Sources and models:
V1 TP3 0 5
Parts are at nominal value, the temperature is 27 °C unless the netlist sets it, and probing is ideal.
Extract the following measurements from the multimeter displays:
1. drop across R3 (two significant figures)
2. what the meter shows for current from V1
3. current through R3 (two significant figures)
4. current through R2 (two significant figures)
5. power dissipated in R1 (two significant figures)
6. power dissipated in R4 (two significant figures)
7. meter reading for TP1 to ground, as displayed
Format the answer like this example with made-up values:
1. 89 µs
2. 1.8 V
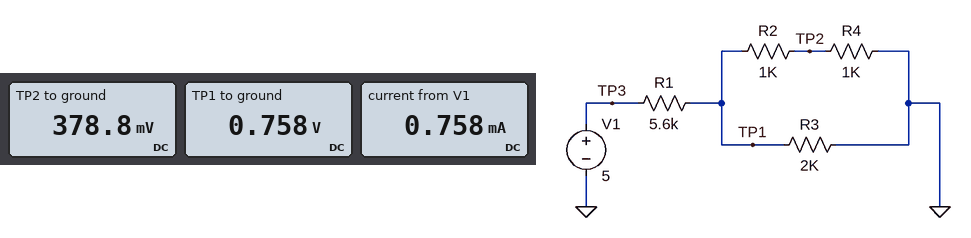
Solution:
1. 760 mV
2. 0.758 mA
3. 380 µA
4. 380 µA
5. 3.2 mW
6. 140 µW
7. 0.758 V
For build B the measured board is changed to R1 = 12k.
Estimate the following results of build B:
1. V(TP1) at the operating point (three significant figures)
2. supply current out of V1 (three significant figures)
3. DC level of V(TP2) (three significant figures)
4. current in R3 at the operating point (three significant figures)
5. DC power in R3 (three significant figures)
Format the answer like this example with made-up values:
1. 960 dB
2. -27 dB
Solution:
1. 385 mV
2. 385 µA
3. 192 mV
4. 192 µA
5. 74.0 µW
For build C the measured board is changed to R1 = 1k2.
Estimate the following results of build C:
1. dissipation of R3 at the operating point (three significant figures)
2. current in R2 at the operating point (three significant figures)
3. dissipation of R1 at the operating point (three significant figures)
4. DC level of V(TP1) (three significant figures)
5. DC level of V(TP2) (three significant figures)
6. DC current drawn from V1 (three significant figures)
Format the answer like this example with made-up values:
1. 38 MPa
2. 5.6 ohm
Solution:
1. 2.58 mW
2. 1.14 mA
3. 6.20 mW
4. 2.27 V
5. 1.14 V
6. 2.27 mA
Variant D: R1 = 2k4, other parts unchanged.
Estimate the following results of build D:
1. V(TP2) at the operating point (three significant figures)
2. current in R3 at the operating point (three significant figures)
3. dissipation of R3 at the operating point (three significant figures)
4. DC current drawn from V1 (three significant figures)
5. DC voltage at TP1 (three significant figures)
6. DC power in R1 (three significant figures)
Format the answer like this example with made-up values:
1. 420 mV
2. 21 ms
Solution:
1. 735 mV
2. 735 µA
3. 1.08 mW
4. 1.47 mA
5. 1.47 V
6. 5.19 mW
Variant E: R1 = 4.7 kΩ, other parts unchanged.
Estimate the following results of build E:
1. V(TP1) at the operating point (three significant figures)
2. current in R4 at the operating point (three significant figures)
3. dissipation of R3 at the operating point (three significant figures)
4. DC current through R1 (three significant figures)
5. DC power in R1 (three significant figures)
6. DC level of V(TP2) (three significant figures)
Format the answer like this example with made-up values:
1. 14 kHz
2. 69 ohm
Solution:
1. 877 mV
2. 439 µA
3. 385 µW
4. 877 µA
5. 3.62 mW
6. 439 mV
